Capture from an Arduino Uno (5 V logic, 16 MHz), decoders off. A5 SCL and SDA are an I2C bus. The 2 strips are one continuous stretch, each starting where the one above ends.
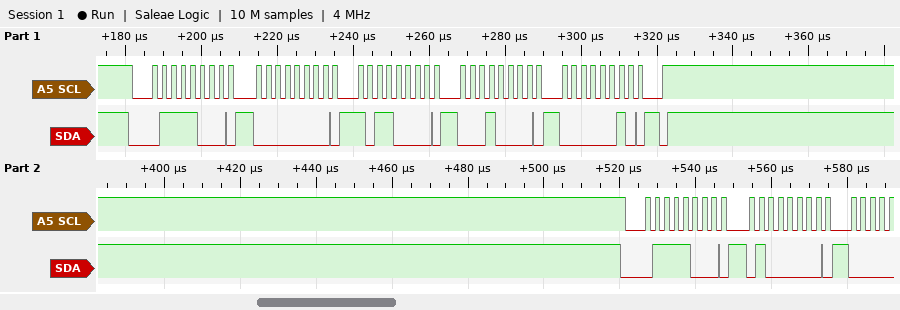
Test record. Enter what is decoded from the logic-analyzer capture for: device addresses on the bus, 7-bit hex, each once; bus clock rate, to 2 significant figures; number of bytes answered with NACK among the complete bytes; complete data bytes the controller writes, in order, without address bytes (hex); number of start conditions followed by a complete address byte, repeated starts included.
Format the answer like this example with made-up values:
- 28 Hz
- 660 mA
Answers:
- 0x3C
- 400 kHz
- 0
- 00 B0 10 02 40
- 2
